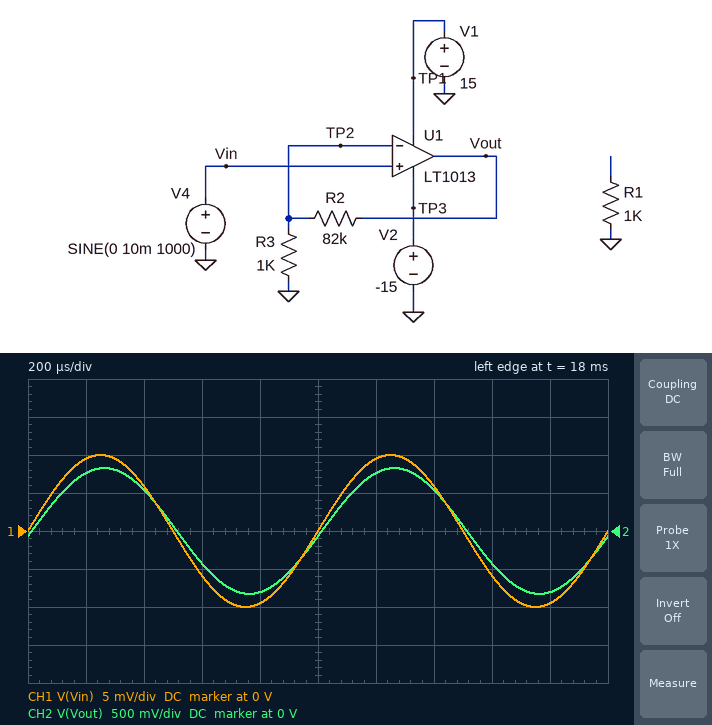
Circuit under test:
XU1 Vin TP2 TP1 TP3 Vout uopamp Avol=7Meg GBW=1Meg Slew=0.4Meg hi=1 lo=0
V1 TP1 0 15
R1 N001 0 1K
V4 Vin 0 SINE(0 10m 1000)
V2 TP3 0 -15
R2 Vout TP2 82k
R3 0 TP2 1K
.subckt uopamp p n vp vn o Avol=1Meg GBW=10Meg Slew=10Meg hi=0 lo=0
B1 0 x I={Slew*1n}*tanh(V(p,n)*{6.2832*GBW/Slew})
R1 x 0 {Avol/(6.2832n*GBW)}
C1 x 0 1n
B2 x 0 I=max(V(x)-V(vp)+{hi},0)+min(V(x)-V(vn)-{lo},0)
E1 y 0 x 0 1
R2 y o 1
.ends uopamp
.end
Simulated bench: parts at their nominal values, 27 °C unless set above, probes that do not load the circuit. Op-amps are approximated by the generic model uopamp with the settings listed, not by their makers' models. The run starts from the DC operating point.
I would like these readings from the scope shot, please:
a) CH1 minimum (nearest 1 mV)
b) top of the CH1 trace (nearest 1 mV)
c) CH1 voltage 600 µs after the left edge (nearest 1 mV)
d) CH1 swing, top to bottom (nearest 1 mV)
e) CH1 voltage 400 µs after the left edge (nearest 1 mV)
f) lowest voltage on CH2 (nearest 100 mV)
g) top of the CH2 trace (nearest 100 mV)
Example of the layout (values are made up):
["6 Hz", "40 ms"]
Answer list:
["-10 mV", "10 mV", "-6 mV", "20 mV", "6 mV", "-800 mV", "800 mV"]
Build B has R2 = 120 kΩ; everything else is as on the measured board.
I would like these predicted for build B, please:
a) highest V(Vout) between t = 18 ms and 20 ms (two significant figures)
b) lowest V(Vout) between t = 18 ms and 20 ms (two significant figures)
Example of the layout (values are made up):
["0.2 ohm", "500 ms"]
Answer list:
["1.2 V", "-1.2 V"]
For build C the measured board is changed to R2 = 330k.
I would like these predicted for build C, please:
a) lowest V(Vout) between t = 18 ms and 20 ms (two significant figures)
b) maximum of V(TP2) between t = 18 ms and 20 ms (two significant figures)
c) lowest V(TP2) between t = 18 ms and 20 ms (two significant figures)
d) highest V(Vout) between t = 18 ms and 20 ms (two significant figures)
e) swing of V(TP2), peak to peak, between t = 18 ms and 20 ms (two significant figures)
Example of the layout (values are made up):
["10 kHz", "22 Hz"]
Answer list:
["-3.1 V", "9.5 mV", "-9.5 mV", "3.1 V", "19 mV"]
